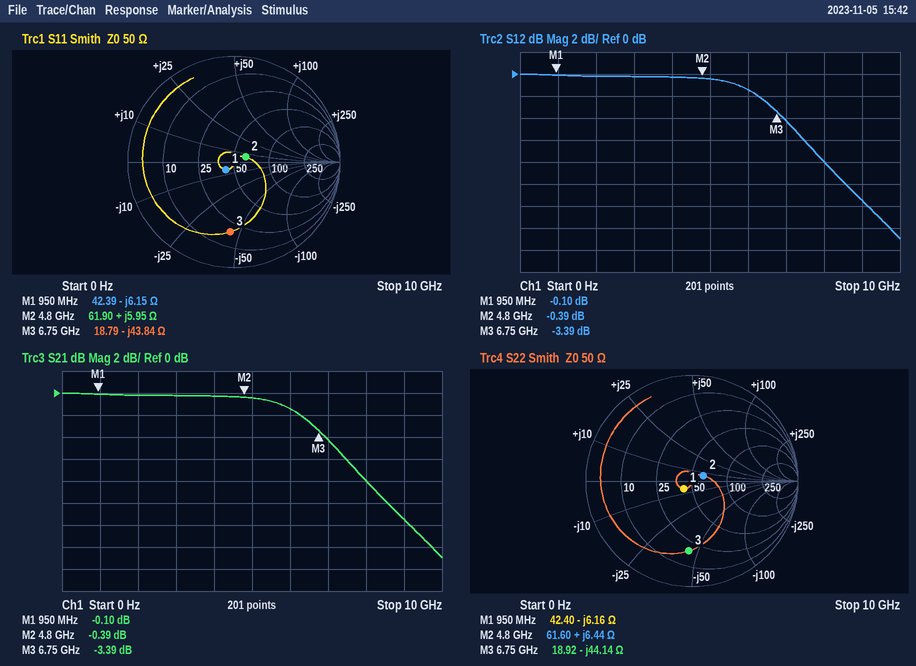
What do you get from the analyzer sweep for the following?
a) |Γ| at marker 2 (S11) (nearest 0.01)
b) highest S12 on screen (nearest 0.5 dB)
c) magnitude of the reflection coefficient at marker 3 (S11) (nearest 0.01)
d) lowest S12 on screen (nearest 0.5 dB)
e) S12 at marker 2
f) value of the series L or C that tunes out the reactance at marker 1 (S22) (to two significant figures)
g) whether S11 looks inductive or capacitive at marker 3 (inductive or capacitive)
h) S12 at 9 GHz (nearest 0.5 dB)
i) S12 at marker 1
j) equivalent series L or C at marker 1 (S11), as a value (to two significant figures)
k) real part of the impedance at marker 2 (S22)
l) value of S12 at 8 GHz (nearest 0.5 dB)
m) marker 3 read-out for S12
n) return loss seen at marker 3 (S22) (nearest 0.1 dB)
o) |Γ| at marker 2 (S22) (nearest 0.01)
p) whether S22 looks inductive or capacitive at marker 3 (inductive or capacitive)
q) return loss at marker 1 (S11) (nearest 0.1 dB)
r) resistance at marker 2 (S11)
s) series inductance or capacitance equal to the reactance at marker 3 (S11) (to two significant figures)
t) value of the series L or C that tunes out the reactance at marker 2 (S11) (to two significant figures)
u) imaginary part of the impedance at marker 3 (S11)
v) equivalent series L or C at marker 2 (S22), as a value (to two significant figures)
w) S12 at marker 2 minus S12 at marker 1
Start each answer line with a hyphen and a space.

- 0.12
- 0.0 dB
- 0.66
- -15.0 dB
- -0.39 dB
- 1.0 nH
- capacitive
- -11.5 dB
- -0.10 dB
- 27 pF
- 61.60 Ω
- -8.0 dB
- -3.39 dB
- 3.6 dB
- 0.12
- capacitive
- 19.5 dB
- 61.90 Ω
- 540 fF
- 5.6 pF
- -43.84 Ω
- 210 pH
- -0.29 dB
